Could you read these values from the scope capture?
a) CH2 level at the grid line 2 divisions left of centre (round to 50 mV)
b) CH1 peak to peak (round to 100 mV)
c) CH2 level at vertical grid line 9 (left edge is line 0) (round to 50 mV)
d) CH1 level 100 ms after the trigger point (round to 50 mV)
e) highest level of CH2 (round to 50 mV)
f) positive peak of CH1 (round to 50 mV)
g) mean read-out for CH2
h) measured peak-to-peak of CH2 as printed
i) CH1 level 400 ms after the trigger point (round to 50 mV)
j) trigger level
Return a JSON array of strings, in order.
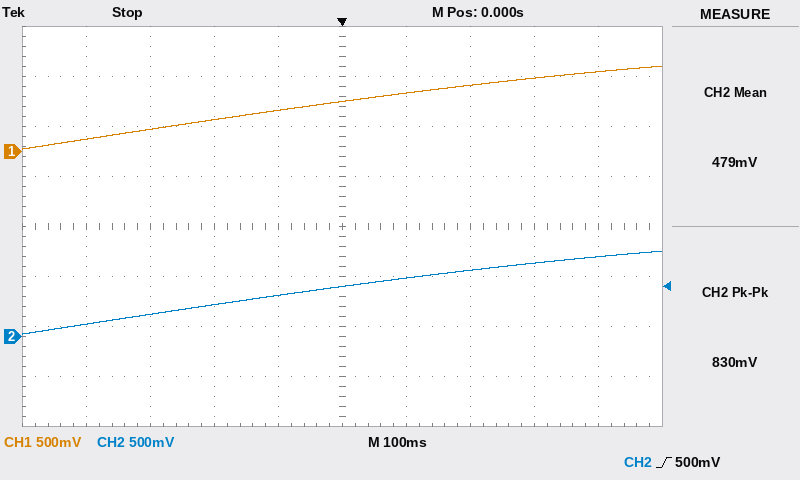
["300 mV", "800 mV", "800 mV", "600 mV", "850 mV", "850 mV", "479 mV", "830 mV", "800 mV", "500 mV"]
